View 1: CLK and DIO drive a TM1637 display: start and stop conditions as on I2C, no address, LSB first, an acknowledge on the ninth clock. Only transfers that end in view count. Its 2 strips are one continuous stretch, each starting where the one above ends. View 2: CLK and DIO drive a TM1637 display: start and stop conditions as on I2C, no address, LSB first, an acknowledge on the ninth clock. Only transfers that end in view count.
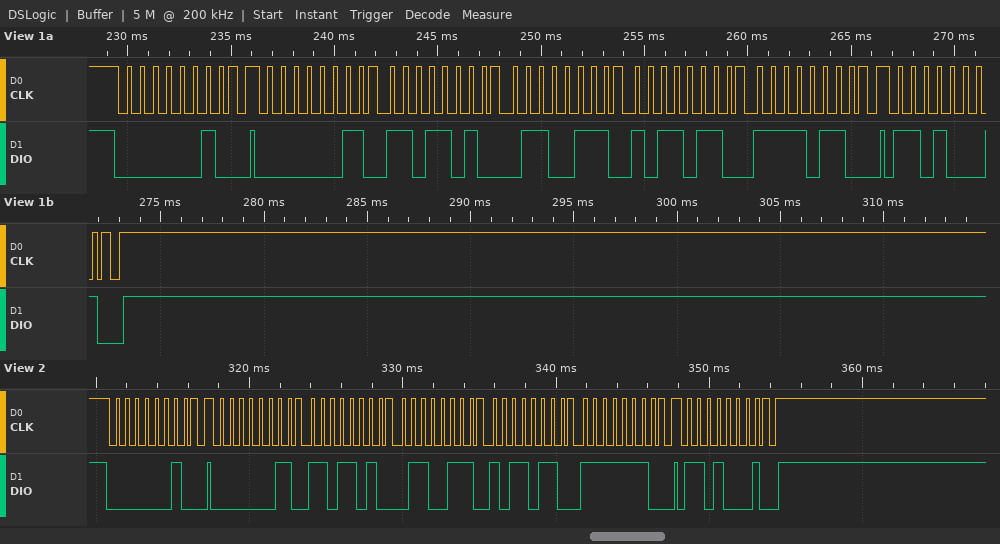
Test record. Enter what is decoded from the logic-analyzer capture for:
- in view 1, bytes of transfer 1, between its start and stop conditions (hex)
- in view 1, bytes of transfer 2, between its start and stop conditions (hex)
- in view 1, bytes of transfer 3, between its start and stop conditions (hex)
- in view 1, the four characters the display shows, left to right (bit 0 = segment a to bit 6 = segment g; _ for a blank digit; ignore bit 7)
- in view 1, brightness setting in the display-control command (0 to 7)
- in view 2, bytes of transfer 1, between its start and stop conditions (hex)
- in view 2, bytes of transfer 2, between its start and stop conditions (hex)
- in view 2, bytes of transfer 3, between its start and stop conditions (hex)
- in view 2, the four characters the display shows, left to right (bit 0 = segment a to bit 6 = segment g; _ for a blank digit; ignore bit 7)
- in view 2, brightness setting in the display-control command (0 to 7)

40
C0 5B E6 6D 6F
8B
2459
3
40
C0 5B E6 6D 7F
8B
2458
3
